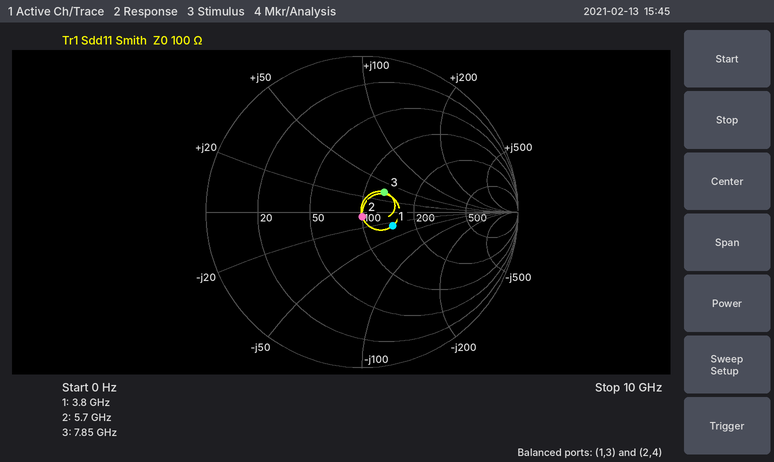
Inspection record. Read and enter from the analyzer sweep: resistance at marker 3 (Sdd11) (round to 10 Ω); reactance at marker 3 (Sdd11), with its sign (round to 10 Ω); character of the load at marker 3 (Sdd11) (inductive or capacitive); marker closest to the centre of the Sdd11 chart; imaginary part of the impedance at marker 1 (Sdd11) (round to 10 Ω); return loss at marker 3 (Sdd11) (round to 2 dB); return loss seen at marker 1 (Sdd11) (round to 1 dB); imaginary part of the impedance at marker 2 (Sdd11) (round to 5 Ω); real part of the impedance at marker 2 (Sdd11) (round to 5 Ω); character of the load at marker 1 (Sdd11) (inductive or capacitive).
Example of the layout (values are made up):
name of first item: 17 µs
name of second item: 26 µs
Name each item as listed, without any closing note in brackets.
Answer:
resistance at marker 3 (Sdd11): 130 Ω
reactance at marker 3 (Sdd11), with its sign: +30 Ω
character of the load at marker 3 (Sdd11): inductive
marker closest to the centre of the Sdd11 chart: marker 2
imaginary part of the impedance at marker 1 (Sdd11): -30 Ω
return loss at marker 3 (Sdd11): 14 dB
return loss seen at marker 1 (Sdd11): 13 dB
imaginary part of the impedance at marker 2 (Sdd11): -5 Ω
real part of the impedance at marker 2 (Sdd11): 100 Ω
character of the load at marker 1 (Sdd11): capacitive
